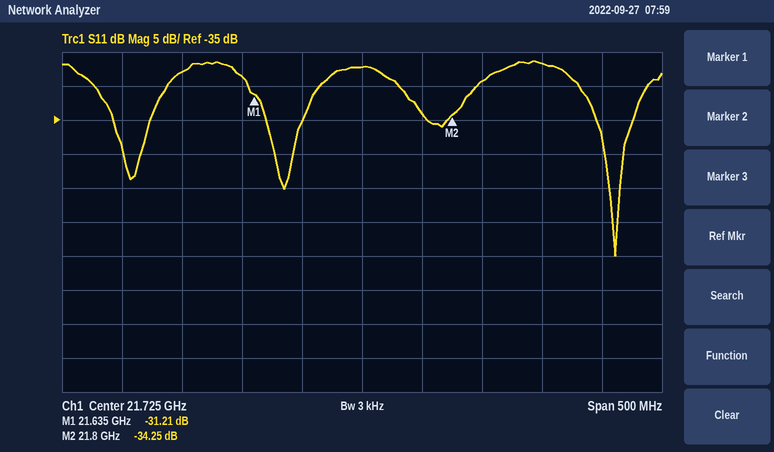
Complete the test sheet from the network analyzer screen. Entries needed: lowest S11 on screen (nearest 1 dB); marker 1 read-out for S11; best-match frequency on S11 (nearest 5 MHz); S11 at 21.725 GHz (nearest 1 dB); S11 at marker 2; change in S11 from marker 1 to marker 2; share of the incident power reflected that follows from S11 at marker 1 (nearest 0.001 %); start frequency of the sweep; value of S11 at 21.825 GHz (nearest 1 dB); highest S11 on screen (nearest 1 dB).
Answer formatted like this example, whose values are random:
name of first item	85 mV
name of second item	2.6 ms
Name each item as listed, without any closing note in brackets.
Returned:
lowest S11 on screen	-55 dB
marker 1 read-out for S11	-31.21 dB
best-match frequency on S11	21.935 GHz
S11 at 21.725 GHz	-27 dB
S11 at marker 2	-34.25 dB
change in S11 from marker 1 to marker 2	-3.04 dB
share of the incident power reflected that follows from S11 at marker 1	0.076 %
start frequency of the sweep	21.475 GHz
value of S11 at 21.825 GHz	-29 dB
highest S11 on screen	-26 dB
